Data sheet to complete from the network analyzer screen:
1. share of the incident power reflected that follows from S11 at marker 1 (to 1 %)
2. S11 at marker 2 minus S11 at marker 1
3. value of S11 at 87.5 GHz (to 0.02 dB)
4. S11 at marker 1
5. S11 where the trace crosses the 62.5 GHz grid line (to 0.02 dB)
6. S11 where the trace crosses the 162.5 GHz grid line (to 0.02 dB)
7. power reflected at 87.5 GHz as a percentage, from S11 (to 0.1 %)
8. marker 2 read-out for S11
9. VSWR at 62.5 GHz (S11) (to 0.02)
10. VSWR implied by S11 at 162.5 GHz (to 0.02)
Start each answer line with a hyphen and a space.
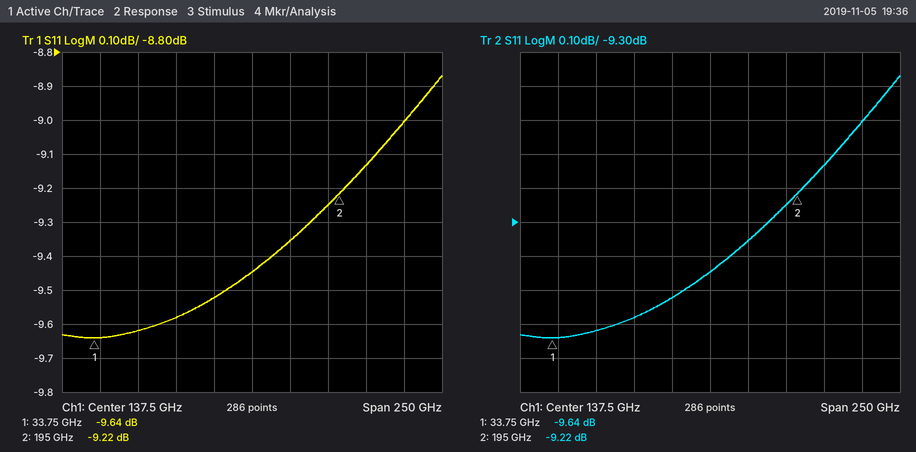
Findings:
- 11 %
- 0.42 dB
- -9.58 dB
- -9.64 dB
- -9.62 dB
- -9.36 dB
- 11.0 %
- -9.22 dB
- 1.98
- 2.04
